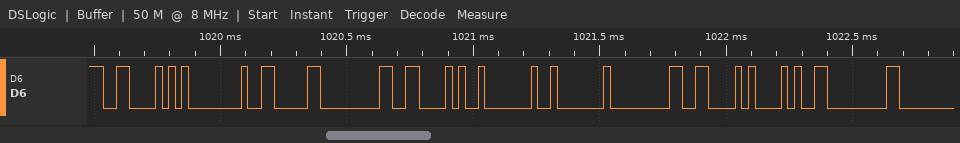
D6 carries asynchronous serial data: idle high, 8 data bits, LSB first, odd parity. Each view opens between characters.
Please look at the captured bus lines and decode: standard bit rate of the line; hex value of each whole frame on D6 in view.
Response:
38400 baud
86, 01, 06, 00, 86, 02, 02, 00, 86, 28, 00
